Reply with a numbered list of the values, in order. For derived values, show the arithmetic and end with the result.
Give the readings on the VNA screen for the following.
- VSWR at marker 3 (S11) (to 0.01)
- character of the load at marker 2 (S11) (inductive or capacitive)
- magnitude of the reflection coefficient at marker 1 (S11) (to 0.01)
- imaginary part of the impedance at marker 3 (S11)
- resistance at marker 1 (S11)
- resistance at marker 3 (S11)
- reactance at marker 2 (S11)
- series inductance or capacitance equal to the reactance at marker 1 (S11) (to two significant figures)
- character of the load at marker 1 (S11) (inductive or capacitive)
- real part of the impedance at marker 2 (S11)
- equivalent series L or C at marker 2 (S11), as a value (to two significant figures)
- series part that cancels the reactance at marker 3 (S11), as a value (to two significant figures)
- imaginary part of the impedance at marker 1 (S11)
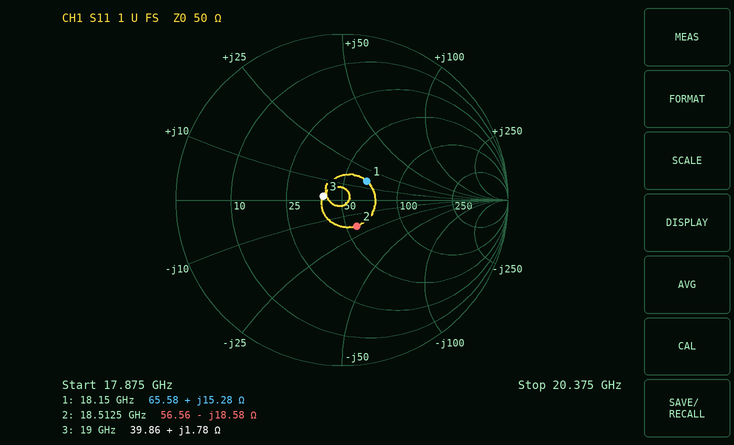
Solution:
1. 1.26
2. capacitive
3. 0.19
4. +1.78 Ω
5. 65.58 Ω
6. 39.86 Ω
7. -18.58 Ω
8. L = 15.28 Ω/(2π × 18.15 GHz) ≈ 134 pH, so 130 pH to two significant figures
9. inductive
10. 56.56 Ω
11. C = 1/(2π × 18.5125 GHz × 18.58 Ω) ≈ 463 fF, so 460 fF to two significant figures
12. C = 1/(2π × 19 GHz × 1.78 Ω) ≈ 4.7 pF
13. +15.28 Ω
